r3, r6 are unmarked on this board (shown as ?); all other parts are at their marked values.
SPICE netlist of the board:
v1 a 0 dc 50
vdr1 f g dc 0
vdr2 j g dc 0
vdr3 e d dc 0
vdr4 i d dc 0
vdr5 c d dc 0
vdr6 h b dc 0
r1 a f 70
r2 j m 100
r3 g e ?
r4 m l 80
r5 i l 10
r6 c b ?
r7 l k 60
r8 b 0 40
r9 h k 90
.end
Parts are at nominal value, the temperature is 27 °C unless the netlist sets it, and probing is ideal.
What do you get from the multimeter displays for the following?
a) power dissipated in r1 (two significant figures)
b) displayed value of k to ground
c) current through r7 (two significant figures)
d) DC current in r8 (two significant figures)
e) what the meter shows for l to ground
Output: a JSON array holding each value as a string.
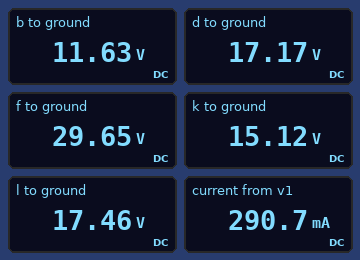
["5.9 W", "15.12 V", "39 mA", "290 mA", "17.46 V"]
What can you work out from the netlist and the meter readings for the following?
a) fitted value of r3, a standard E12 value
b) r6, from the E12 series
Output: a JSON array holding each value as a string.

["56 Ω", "22 Ω"]
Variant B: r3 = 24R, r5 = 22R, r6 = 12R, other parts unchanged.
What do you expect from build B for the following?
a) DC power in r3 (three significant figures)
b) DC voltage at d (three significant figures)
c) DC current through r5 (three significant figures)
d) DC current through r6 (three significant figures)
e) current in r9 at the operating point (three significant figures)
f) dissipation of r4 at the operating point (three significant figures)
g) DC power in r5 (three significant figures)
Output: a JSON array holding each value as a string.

["2.33 W", "17.9 V", "12.3 mA", "324 mA", "27.7 mA", "128 mW", "3.33 mW"]
